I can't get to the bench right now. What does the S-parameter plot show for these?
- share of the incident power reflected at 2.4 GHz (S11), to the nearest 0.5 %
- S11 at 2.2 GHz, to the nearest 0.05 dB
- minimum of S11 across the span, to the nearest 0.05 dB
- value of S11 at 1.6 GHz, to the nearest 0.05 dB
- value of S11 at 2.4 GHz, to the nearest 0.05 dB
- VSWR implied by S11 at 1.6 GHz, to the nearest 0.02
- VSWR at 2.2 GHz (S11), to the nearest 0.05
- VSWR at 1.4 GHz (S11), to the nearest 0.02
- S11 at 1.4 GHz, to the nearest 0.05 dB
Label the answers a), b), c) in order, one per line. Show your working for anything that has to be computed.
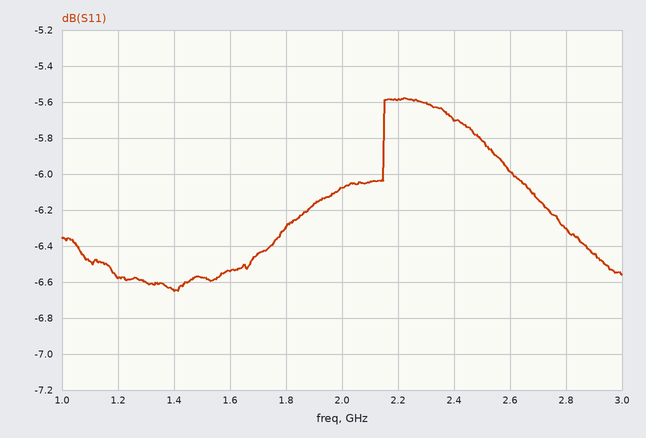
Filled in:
a) 10^(-5.7/10) ≈ 26.9 %, so 27.0 % to the nearest 0.5 %
b) -5.60 dB
c) -6.65 dB
d) -6.55 dB
e) -5.70 dB
f) |Γ| = 10^(-6.55/20) = 0.4704; VSWR = (1 + 0.4704)/(1 − 0.4704) ≈ 2.78
g) |Γ| = 10^(-5.6/20) = 0.5248; VSWR = (1 + 0.5248)/(1 − 0.5248) ≈ 3.21, so 3.20 to the nearest 0.05
h) |Γ| = 10^(-6.65/20) = 0.4651; VSWR = (1 + 0.4651)/(1 − 0.4651) ≈ 2.74
i) -6.65 dB
